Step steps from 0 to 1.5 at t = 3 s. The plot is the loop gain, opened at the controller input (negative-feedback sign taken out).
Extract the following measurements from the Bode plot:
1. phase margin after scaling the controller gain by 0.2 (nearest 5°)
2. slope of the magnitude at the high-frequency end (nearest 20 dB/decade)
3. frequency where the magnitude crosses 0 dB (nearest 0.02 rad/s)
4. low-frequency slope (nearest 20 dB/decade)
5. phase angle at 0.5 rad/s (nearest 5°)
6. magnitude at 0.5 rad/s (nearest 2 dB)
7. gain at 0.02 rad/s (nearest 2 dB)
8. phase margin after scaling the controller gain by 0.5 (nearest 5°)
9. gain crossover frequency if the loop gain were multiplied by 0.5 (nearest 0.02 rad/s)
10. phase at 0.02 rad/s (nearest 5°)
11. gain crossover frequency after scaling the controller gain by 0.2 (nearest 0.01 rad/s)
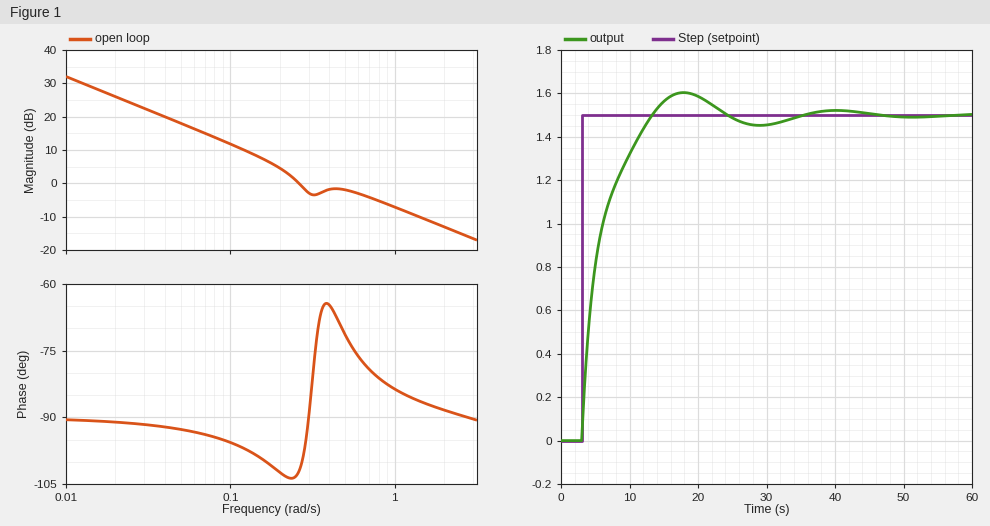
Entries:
85°
-20 dB/decade
0.26 rad/s
-20 dB/decade
-70°
-2 dB
26 dB
80°
0.18 rad/s
-90°
0.08 rad/s
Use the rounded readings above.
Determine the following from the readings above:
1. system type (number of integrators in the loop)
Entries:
1
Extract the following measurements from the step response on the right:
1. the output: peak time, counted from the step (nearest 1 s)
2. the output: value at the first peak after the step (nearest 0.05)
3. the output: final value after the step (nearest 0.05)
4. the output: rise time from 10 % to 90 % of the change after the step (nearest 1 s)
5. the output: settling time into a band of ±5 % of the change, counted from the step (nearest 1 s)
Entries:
15 s
1.60
1.50
7 s
18 s
